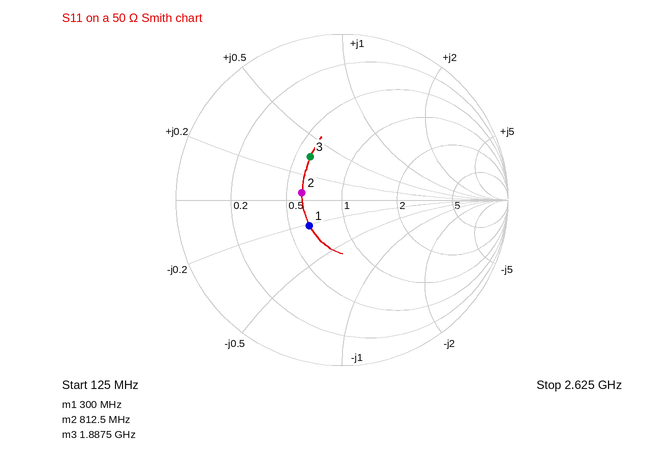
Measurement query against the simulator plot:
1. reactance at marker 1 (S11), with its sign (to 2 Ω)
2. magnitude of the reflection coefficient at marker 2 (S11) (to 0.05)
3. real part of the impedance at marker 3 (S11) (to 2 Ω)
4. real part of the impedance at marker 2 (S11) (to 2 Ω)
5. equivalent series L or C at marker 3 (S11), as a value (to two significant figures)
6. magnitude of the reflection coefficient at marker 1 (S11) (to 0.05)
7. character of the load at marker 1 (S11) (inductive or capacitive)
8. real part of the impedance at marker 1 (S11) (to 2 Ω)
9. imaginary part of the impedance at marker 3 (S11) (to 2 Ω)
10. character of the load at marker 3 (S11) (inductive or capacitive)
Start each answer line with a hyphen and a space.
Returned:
- -10 Ω
- 0.25
- 30 Ω
- 30 Ω
- 1.5 nH
- 0.25
- capacitive
- 32 Ω
- +18 Ω
- inductive
